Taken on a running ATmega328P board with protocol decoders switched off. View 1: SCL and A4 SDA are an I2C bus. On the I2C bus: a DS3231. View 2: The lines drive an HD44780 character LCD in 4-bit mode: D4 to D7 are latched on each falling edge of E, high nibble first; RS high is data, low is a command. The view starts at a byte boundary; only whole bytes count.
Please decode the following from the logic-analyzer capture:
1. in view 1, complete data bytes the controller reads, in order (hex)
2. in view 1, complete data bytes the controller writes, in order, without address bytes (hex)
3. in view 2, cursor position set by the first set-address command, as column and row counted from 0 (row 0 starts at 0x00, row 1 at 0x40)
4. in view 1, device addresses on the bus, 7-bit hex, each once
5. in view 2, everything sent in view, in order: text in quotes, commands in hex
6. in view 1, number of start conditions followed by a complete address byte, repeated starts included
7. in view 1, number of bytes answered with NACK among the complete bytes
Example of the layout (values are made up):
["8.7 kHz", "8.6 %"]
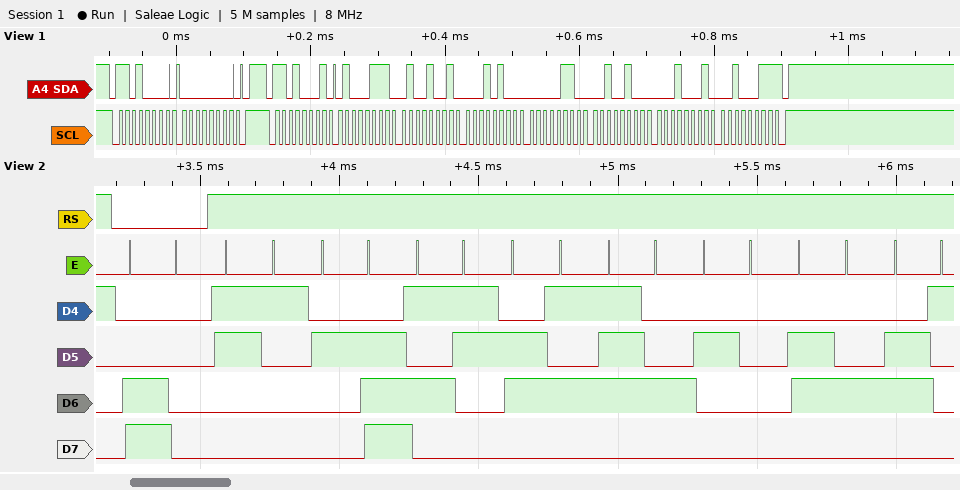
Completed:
["47 49 14 06 24 11 23", "00", "column 0, row 1", "0x68", "0xC0 \"1.Set da\"", "2", "1"]
